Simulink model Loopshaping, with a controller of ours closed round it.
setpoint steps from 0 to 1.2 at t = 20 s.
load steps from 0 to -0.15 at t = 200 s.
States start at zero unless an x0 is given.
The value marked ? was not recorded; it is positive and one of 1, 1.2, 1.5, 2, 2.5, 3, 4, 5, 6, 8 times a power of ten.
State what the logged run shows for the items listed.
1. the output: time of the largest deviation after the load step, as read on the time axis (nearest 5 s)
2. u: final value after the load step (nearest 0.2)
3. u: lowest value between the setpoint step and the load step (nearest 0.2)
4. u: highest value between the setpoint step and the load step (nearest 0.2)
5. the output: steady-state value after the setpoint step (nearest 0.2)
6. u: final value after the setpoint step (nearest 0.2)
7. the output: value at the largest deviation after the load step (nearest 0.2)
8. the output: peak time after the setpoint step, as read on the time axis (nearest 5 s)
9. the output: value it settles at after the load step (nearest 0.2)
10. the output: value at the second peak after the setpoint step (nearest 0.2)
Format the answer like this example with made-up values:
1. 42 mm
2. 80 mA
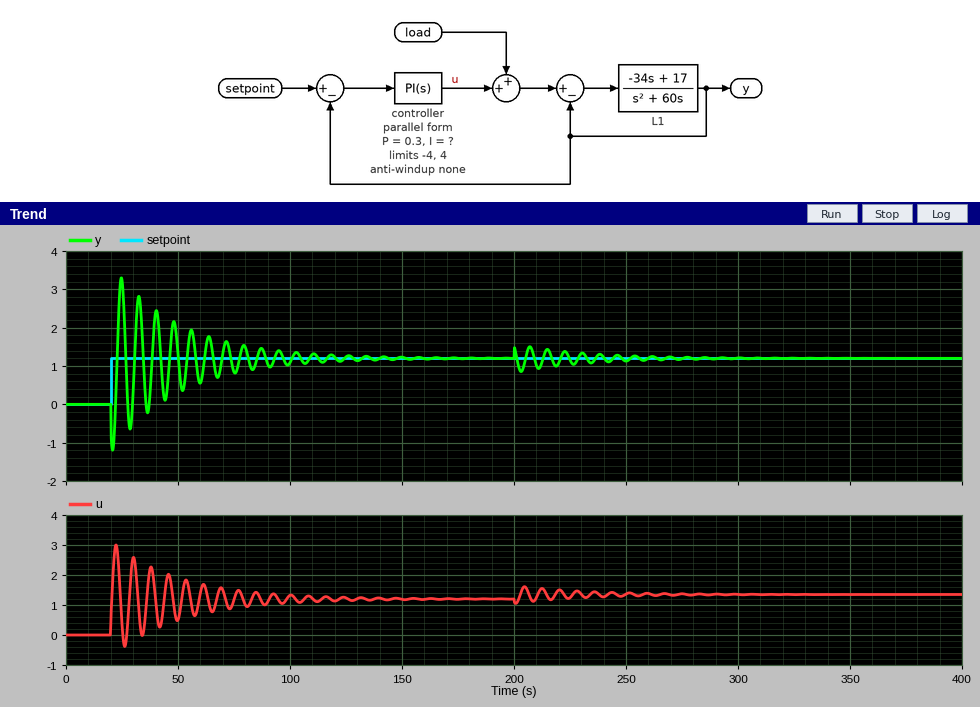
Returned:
1. 205 s
2. 1.4
3. -0.4
4. 3.0
5. 1.2
6. 1.2
7. 0.8
8. 25 s
9. 1.2
10. 2.8
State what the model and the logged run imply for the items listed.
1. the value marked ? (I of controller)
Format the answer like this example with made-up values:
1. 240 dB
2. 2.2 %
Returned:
1. 0.6
